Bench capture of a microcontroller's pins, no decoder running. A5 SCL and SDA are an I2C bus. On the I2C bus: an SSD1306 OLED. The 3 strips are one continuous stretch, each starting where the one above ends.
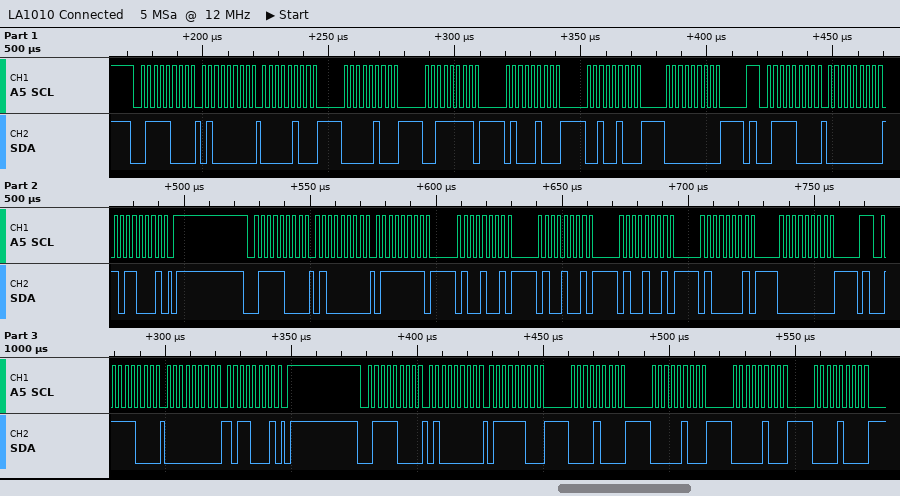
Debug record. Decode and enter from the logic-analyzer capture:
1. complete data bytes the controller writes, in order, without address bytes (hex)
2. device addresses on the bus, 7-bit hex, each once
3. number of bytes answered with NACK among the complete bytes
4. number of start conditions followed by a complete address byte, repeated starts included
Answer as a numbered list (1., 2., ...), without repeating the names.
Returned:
1. 40 04 04 3F 44 24 00 00 B1 40 7F 49 49 49 41 00 00 B1 40 7C 08 04 04 08
2. 0x3C
3. 0
4. 5
